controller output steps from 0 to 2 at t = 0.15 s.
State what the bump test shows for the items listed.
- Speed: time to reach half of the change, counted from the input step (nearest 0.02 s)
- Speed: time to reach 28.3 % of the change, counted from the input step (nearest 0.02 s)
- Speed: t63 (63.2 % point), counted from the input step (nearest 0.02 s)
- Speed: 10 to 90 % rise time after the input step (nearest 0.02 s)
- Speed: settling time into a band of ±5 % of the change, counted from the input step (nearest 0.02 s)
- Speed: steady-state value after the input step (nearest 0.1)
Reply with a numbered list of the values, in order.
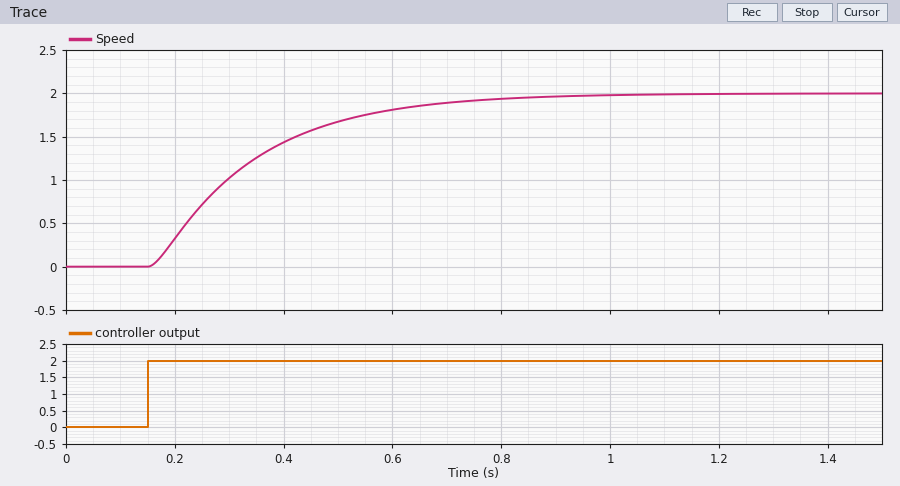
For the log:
1. 0.14 s
2. 0.08 s
3. 0.20 s
4. 0.40 s
5. 0.56 s
6. 2.0
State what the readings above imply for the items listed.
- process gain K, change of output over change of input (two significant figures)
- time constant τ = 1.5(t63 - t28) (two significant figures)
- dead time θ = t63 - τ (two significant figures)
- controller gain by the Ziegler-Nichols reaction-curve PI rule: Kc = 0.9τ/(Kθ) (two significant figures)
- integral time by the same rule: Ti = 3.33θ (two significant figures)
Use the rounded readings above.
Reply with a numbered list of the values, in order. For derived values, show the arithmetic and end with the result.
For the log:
1. (2 - 0) / 2 = 1.0
2. 1.5 × (0.2 - 0.08) = 0.18 s
3. 0.2 - 0.18 = 0.020 s
4. 0.9 × 0.18 / (1 × 0.02) = 8.1
5. 3.33 × 0.02 = 0.067 s
